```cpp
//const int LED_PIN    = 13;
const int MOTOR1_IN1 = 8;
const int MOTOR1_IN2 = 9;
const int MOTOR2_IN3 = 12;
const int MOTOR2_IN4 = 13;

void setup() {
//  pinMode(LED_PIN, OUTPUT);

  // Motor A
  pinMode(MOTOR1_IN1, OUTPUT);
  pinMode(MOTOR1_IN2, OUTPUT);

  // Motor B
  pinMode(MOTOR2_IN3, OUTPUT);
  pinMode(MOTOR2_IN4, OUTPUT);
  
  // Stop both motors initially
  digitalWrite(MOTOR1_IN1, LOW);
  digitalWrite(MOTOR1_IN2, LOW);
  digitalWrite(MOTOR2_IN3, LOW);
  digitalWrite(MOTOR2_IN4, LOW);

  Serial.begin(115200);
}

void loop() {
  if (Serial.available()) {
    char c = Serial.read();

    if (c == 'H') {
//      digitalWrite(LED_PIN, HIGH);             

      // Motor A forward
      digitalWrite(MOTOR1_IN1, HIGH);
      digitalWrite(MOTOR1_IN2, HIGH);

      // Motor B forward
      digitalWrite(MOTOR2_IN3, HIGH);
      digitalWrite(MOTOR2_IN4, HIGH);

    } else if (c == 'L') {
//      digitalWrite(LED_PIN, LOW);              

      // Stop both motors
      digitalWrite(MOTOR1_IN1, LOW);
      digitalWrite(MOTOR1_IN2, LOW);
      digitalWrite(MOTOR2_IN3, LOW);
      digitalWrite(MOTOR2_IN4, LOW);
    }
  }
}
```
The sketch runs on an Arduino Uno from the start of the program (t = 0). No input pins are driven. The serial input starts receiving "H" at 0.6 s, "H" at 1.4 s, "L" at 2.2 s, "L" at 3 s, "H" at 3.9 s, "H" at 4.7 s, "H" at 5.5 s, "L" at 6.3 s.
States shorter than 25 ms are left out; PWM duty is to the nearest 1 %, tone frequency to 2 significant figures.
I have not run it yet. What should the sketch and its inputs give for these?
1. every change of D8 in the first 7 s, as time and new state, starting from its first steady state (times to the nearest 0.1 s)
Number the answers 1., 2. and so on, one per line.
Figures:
1. 0 s low; 0.6 s high; 2.2 s low; 3.9 s high; 6.3 s low
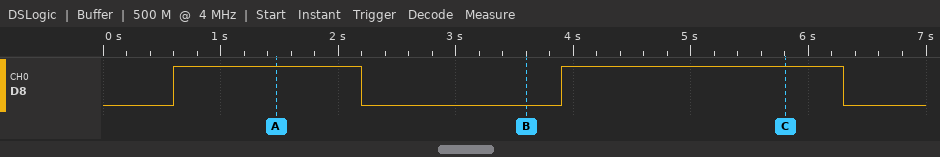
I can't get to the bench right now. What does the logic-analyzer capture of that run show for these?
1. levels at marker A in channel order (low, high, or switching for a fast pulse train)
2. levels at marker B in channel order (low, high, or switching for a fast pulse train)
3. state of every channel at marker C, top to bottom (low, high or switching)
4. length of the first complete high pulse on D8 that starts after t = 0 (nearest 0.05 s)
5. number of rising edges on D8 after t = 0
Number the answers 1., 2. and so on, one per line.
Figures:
1. D8 high
2. D8 low
3. D8 high
4. 1.60 s
5. 2
